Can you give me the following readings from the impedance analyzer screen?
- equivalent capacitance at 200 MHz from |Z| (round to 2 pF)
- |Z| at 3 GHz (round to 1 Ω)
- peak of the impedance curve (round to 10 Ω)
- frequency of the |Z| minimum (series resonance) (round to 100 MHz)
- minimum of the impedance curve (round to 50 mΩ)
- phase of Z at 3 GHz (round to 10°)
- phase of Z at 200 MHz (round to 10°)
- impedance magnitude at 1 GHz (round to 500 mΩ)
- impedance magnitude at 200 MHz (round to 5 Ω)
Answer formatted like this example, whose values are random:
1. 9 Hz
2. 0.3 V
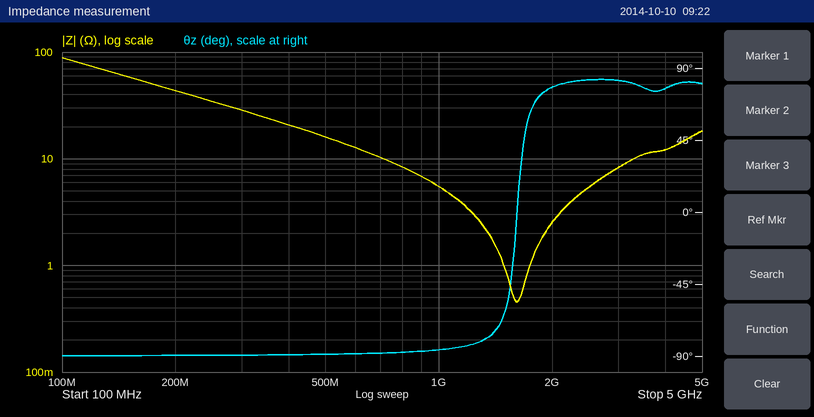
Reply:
1. 18 pF
2. 8 Ω
3. 90 Ω
4. 1.6 GHz
5. 450 mΩ
6. 80°
7. -90°
8. 5.5 Ω
9. 45 Ω
